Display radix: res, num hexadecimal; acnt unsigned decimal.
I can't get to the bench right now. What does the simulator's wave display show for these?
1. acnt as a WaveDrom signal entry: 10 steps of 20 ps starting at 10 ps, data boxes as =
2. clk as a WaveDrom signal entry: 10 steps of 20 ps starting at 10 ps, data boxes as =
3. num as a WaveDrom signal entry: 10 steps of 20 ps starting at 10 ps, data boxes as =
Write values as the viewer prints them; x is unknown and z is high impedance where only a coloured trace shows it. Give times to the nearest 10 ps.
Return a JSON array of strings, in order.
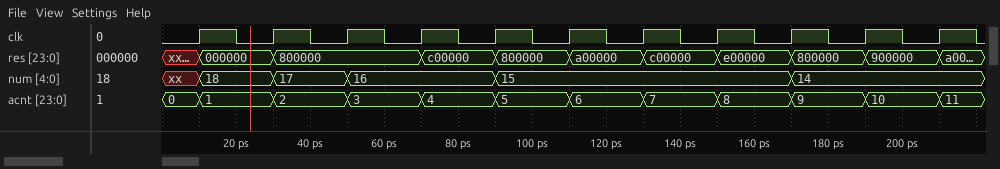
["{name: 'acnt', wave: '==========', data: '1 2 3 4 5 6 7 8 9 10'}", "{name: 'clk', wave: 'p.........'}", "{name: 'num', wave: '===.=...=.', data: '18 17 16 15 14'}"]
